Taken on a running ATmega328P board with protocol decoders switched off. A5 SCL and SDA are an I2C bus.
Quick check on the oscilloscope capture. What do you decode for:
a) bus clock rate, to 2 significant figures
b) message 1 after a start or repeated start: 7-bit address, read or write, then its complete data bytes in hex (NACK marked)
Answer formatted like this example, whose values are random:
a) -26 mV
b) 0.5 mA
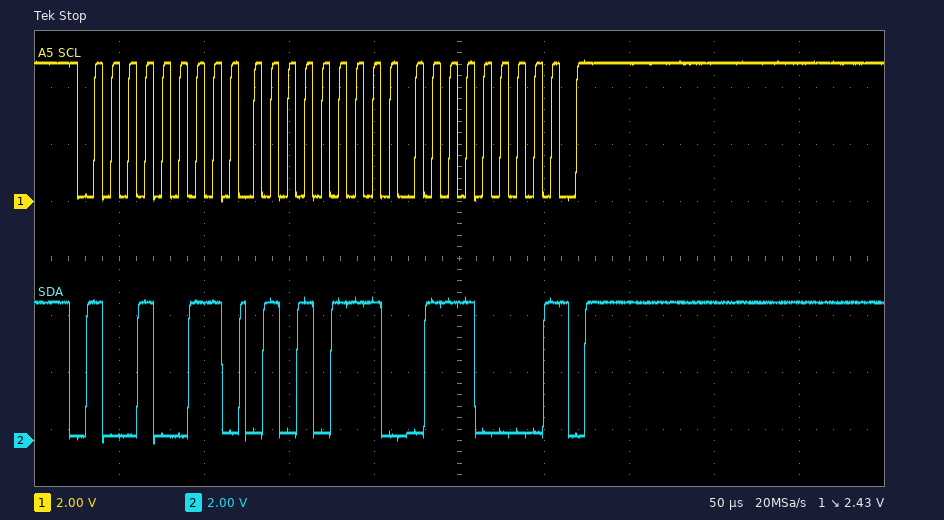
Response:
a) 100 kHz
b) 0x49 read: 57 70 NACK
